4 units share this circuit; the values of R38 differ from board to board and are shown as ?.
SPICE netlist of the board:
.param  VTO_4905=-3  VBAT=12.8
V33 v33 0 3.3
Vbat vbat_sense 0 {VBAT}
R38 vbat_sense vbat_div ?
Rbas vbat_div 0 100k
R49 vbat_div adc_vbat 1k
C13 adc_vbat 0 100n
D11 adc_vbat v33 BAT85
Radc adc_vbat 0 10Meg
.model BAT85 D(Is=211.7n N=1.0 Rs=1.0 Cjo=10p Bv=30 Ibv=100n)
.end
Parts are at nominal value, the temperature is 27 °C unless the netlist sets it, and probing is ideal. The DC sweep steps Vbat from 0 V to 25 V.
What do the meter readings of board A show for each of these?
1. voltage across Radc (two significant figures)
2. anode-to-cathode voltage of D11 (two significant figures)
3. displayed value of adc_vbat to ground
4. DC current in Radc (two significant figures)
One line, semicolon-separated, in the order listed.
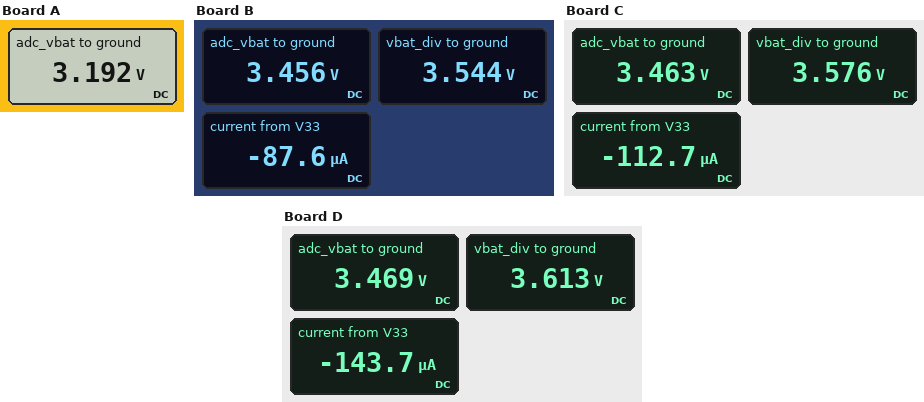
3.2 V; -110 mV; 3.192 V; 320 nA
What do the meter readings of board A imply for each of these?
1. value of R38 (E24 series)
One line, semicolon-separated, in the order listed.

300 kΩ
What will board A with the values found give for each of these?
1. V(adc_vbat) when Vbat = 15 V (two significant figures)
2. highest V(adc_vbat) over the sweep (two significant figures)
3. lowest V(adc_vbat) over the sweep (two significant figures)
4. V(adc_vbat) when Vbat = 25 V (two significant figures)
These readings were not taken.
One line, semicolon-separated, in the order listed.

3.4 V; 3.4 V; 16 mV; 3.4 V
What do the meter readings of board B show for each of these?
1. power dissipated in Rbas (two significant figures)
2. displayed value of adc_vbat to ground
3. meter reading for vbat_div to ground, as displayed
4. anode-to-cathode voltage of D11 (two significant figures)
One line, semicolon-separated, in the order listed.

130 µW; 3.456 V; 3.544 V; 160 mV
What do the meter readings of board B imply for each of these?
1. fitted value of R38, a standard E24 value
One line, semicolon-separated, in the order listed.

75 kΩ
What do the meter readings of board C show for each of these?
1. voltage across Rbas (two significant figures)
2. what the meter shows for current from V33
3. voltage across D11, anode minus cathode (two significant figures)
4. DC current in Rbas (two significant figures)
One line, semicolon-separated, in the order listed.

3.6 V; -112.7 µA; 160 mV; 36 µA
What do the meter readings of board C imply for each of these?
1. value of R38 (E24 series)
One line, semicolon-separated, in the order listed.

62 kΩ
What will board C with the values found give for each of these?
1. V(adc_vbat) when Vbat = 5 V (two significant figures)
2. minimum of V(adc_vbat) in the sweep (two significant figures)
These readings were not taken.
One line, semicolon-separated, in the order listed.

3.1 V; 8.3 mV
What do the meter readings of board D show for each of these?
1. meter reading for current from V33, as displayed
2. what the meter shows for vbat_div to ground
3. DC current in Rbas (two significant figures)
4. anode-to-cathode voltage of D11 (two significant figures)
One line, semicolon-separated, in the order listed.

-143.7 µA; 3.613 V; 36 µA; 170 mV
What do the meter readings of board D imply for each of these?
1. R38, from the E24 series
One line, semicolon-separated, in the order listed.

51 kΩ
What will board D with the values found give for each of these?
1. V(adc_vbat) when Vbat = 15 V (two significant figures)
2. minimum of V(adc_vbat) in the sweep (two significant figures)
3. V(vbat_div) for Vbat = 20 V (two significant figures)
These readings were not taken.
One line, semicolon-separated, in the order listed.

3.5 V; 7.3 mV; 3.8 V
